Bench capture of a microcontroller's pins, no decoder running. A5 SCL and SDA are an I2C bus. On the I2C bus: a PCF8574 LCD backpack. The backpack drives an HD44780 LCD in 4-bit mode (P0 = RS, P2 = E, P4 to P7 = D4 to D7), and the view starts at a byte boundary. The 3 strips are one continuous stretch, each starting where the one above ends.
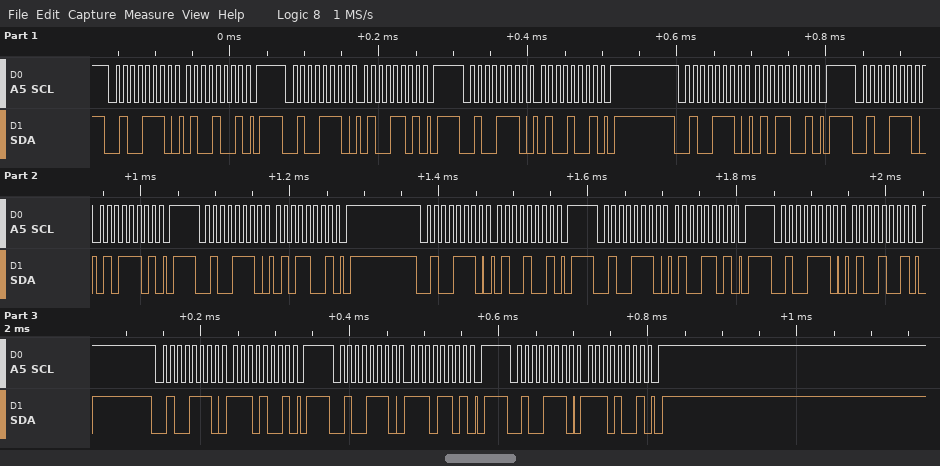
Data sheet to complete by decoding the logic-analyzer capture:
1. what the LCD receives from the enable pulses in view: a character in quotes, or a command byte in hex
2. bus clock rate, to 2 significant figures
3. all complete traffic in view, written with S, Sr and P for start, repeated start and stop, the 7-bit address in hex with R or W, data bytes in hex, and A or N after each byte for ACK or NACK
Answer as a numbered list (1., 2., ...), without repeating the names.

1. 'E' 'N'
2. 100 kHz
3. S 27W A 49 A P S 27W A 4D A P S 27W A 49 A P S 27W A 59 A P S 27W A 5D A P S 27W A 59 A P S 27W A 49 A P S 27W A 4D A P S 27W A 49 A P S 27W A E9 A P S 27W A ED A P S 27W A E9 A P
